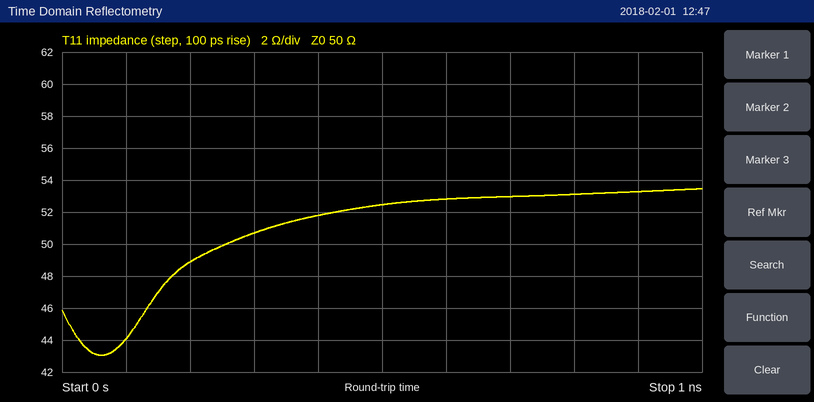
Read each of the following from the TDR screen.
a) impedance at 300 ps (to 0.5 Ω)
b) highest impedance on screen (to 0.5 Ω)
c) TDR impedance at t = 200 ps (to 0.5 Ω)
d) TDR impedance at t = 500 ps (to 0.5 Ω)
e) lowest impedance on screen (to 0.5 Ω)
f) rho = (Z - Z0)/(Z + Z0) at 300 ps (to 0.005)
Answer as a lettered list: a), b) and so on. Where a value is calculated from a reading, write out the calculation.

a) 50.5 Ω
b) 53.5 Ω
c) 49.0 Ω
d) 52.5 Ω
e) 43.0 Ω
f) (50.5 − 50)/(50.5 + 50) ≈ +0.005
